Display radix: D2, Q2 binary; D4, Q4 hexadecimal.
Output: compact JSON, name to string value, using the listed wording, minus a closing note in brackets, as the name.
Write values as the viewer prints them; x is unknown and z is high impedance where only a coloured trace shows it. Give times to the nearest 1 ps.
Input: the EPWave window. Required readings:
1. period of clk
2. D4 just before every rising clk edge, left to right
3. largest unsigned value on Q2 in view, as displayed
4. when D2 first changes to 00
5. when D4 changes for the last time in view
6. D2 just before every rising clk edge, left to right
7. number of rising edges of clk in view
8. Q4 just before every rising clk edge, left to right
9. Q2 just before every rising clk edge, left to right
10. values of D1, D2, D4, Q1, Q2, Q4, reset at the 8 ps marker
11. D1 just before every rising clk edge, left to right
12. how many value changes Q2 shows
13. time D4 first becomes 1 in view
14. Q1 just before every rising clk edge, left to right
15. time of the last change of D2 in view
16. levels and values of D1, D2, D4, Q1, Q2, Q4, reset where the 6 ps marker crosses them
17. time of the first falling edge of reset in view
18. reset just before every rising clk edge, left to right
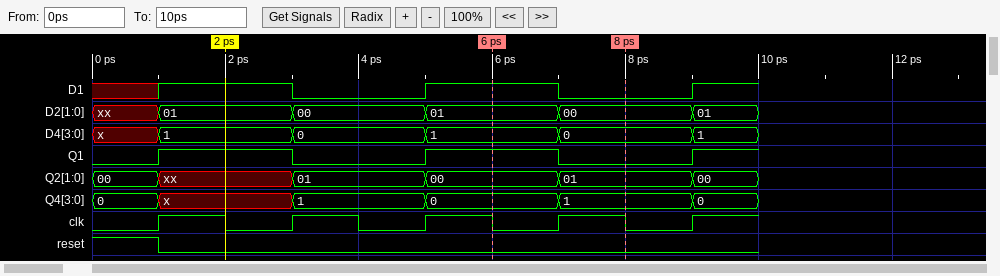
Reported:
{"period of clk": "2 ps", "D4 just before every rising clk edge, left to right": "x, 1, 0, 1, 0", "largest unsigned value on Q2 in view, as displayed": "01", "when D2 first changes to 00": "3 ps", "when D4 changes for the last time in view": "9 ps", "D2 just before every rising clk edge, left to right": "xx, 01, 00, 01, 00", "number of rising edges of clk in view": "5", "Q4 just before every rising clk edge, left to right": "0, x, 1, 0, 1", "Q2 just before every rising clk edge, left to right": "00, xx, 01, 00, 01", "values of D1, D2, D4, Q1, Q2, Q4, reset at the 8 ps marker": "D1=0, D2=00, D4=0, Q1=0, Q2=01, Q4=1, reset=0", "D1 just before every rising clk edge, left to right": "x 1 0 1 0", "how many value changes Q2 shows": "5", "time D4 first becomes 1 in view": "1 ps", "Q1 just before every rising clk edge, left to right": "0 1 0 1 0", "time of the last change of D2 in view": "9 ps", "levels and values of D1, D2, D4, Q1, Q2, Q4, reset where the 6 ps marker crosses them": "D1=1, D2=01, D4=1, Q1=1, Q2=00, Q4=0, reset=0", "time of the first falling edge of reset in view": "1 ps", "reset just before every rising clk edge, left to right": "1 0 0 0 0"}
